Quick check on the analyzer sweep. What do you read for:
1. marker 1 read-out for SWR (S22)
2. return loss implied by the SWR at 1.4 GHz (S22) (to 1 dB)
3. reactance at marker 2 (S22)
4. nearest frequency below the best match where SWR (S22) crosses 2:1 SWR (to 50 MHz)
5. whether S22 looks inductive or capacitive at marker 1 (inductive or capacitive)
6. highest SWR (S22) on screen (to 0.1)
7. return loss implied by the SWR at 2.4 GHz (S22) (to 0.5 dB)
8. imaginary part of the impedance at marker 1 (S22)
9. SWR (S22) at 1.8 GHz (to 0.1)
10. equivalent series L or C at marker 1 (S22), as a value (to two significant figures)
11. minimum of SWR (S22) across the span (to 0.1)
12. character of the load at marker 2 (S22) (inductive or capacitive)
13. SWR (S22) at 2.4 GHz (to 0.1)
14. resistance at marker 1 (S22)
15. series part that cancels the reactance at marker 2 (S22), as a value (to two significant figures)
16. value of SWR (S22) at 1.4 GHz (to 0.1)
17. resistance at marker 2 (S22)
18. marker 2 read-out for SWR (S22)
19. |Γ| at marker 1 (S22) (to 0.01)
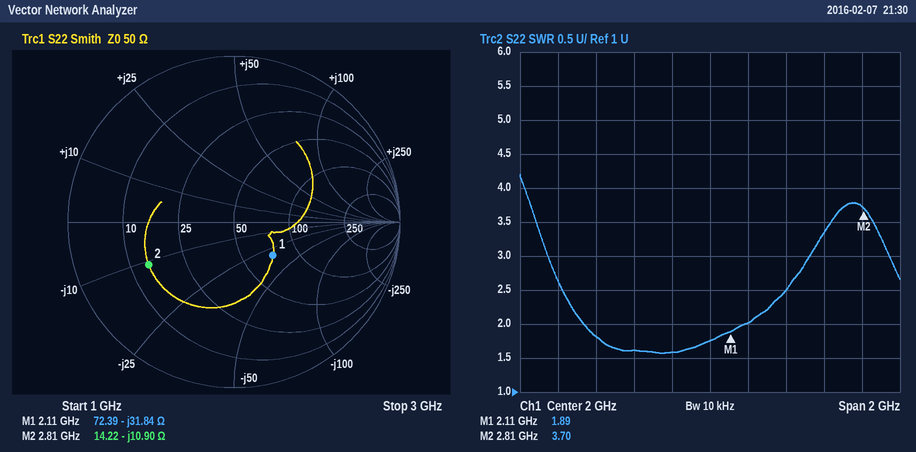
1.89
11 dB
-10.90 Ω
1.35 GHz
capacitive
4.2
7.5 dB
-31.84 Ω
1.6
2.4 pF
1.6
capacitive
2.5
72.39 Ω
620 pH
1.8
14.22 Ω
3.70
0.31
